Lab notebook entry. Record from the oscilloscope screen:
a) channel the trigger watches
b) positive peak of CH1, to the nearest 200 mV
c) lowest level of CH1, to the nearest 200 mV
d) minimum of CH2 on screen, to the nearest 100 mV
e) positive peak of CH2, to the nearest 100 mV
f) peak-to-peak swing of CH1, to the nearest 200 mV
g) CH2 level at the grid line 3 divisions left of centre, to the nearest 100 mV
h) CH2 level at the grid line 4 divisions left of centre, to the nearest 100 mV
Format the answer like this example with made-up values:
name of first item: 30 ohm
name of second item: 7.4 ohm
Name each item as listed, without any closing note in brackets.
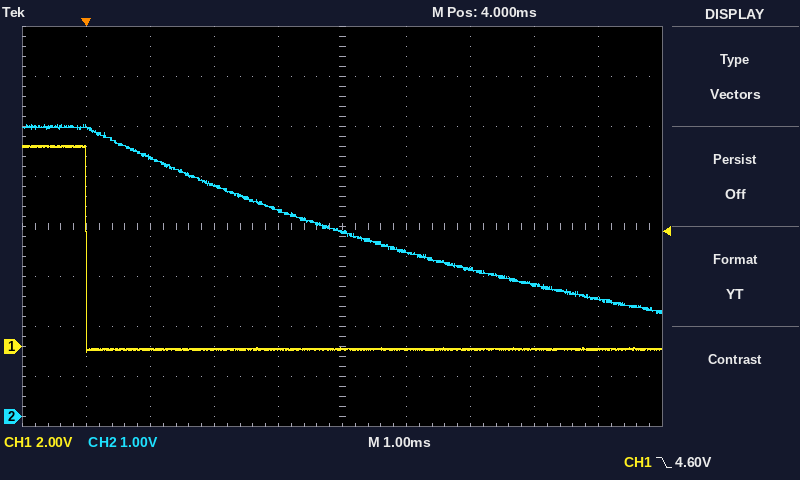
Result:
channel the trigger watches: CH1
positive peak of CH1, to the nearest 200 mV: 8.0 V
lowest level of CH1, to the nearest 200 mV: -200 mV
minimum of CH2 on screen, to the nearest 100 mV: 2.1 V
positive peak of CH2, to the nearest 100 mV: 5.8 V
peak-to-peak swing of CH1, to the nearest 200 mV: 8.2 V
CH2 level at the grid line 3 divisions left of centre, to the nearest 100 mV: 5.2 V
CH2 level at the grid line 4 divisions left of centre, to the nearest 100 mV: 5.8 V
